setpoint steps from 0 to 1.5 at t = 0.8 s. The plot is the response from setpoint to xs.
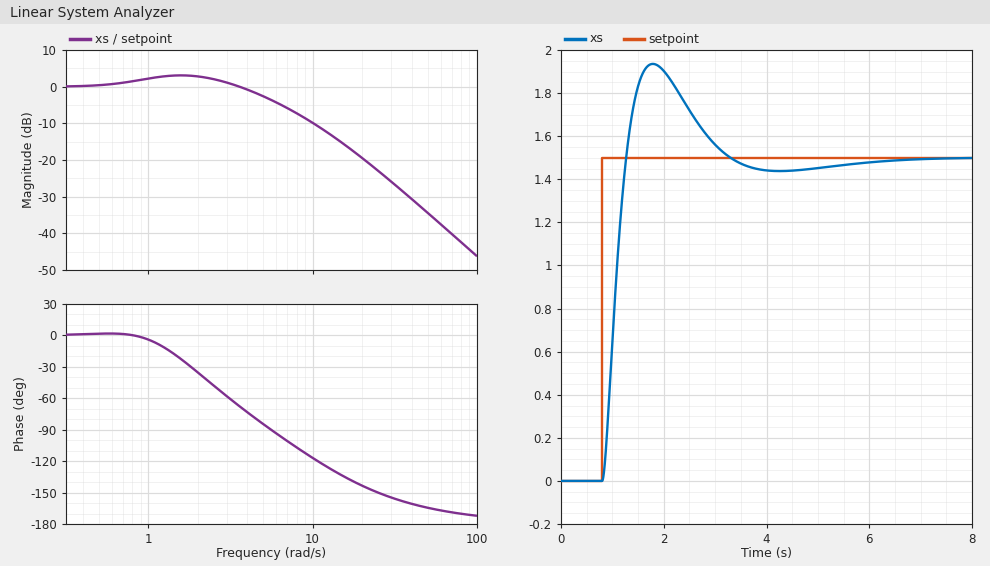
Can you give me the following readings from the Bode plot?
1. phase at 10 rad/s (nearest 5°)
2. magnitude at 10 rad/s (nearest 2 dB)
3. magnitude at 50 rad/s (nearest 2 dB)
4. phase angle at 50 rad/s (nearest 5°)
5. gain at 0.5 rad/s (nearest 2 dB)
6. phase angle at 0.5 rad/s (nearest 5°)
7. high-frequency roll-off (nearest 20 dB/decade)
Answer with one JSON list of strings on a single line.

["-115°", "-10 dB", "-34 dB", "-165°", "0 dB", "0°", "-40 dB/decade"]
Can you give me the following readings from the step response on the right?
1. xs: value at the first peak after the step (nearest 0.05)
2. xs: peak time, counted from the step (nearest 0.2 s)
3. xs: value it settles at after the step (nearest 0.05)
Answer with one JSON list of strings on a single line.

["1.95", "1.0 s", "1.50"]
